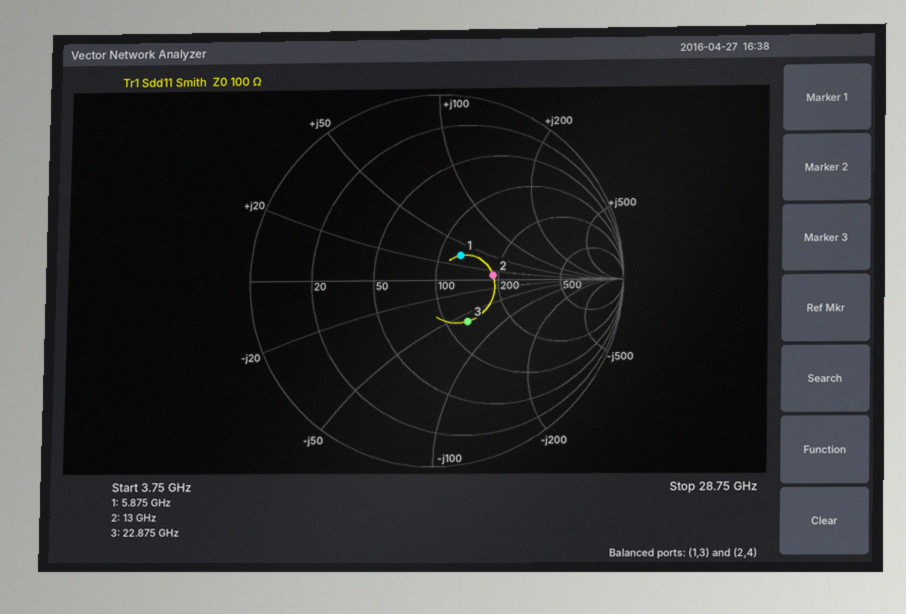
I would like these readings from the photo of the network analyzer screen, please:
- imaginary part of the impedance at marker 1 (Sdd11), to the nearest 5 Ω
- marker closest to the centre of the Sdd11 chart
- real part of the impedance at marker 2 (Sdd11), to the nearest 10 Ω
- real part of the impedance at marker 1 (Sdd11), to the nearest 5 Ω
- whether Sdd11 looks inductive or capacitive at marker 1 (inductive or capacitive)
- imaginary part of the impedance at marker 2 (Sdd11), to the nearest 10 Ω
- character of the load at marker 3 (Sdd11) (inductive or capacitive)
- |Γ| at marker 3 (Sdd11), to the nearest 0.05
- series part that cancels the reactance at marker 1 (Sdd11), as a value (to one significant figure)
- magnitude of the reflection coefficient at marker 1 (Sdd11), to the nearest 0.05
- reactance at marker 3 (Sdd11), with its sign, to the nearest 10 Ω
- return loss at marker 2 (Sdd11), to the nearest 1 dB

+35 Ω
marker 1
190 Ω
125 Ω
inductive
+10 Ω
capacitive
0.30
800 fF
0.20
-60 Ω
10 dB
